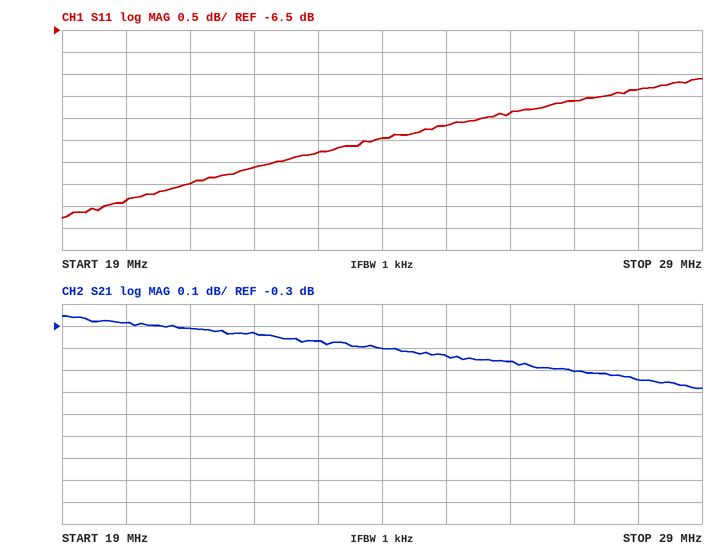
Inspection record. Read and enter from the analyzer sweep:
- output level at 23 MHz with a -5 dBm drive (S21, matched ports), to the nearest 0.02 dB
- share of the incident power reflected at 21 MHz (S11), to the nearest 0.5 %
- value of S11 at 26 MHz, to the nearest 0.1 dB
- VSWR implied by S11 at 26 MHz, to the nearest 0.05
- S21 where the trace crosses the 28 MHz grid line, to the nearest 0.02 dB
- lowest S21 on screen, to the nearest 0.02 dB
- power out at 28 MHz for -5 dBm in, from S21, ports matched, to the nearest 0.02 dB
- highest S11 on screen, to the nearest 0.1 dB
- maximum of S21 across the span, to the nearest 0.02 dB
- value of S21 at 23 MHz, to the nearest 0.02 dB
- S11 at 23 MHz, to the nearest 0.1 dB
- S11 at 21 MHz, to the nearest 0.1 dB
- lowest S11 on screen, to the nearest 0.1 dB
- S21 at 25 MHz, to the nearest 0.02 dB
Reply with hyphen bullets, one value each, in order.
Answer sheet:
- -5.36 dBm
- 10.0 %
- -8.4 dB
- 2.25
- -0.54 dB
- -0.58 dB
- -5.54 dBm
- -7.6 dB
- -0.26 dB
- -0.36 dB
- -9.3 dB
- -10.0 dB
- -10.8 dB
- -0.44 dB
